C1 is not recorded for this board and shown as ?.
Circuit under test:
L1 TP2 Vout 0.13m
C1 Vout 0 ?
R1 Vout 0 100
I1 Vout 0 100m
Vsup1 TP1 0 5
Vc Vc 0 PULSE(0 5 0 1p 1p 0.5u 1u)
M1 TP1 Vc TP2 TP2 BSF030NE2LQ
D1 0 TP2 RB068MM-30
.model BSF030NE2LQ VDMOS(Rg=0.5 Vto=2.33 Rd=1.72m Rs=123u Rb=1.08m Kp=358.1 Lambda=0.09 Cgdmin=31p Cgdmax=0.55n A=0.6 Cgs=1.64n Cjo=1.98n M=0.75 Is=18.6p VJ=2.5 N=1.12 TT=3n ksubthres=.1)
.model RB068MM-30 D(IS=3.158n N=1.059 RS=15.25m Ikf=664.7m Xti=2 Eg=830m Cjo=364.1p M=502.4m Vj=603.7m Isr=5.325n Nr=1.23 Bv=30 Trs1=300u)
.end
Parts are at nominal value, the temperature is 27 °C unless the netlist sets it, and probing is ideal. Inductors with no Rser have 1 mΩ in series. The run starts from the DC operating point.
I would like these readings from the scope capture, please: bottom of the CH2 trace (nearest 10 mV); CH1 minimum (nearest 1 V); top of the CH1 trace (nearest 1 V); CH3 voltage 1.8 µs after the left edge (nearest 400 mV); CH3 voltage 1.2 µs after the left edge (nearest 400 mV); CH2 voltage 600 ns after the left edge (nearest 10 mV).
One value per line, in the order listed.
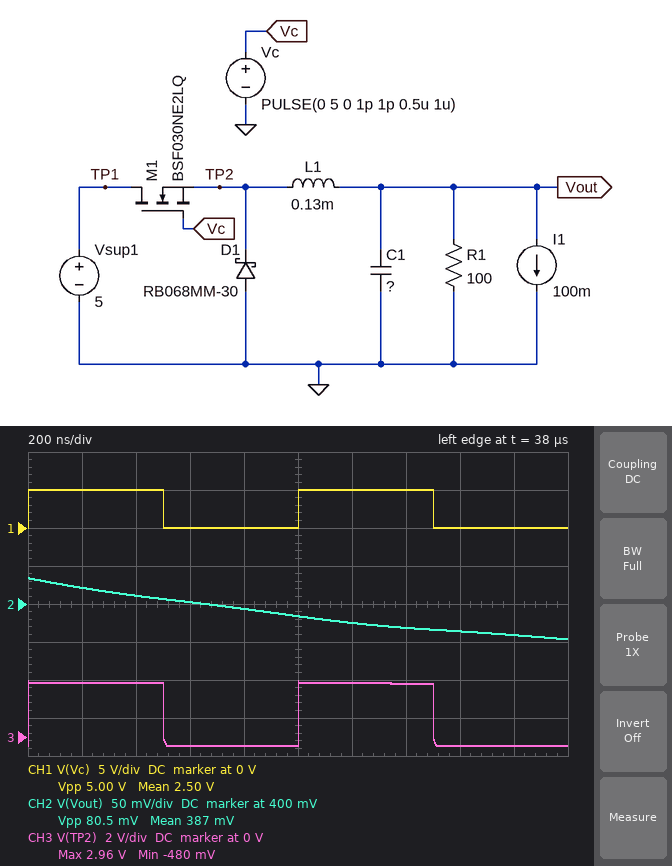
350 mV
0 V
5 V
-400 mV
2.8 V
400 mV
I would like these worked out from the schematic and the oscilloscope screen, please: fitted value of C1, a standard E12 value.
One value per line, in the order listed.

330 nF
